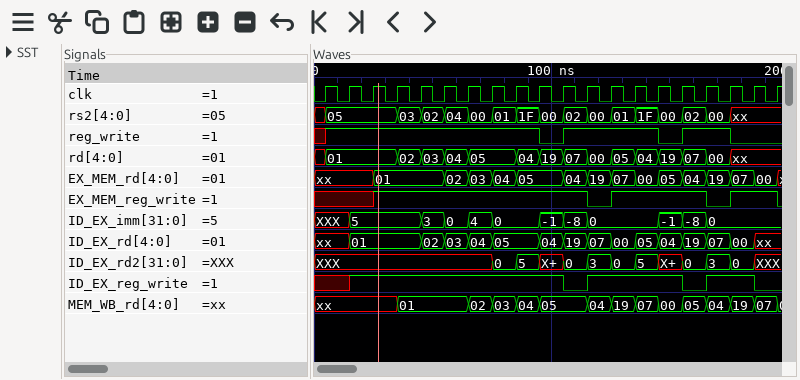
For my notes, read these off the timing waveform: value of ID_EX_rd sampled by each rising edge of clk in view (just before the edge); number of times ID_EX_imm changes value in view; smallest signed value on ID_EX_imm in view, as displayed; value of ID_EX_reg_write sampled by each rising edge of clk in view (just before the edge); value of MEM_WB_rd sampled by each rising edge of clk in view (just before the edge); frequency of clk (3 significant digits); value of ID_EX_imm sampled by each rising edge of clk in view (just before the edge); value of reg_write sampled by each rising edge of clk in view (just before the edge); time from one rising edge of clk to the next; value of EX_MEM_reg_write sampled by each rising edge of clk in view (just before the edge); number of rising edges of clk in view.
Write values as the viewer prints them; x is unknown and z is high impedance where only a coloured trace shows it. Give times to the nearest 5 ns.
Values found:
xx, xx, 01, 01, 01, 02, 03, 04, 05, 05, 04, 19, 07, 00, 05, 04, 19, 07, 00, xx
11
-8
x x 1 1 1 1 1 1 1 1 1 0 1 1 1 1 0 1 1 0
xx, xx, xx, xx, 01, 01, 01, 02, 03, 04, 05, 05, 04, 19, 07, 00, 05, 04, 19, 07
100 MHz
XXX, XXX, 5, 5, 5, 3, 0, 4, 0, 0, -1, -8, 0, 0, 0, -1, -8, 0, 0, 0
x 1 1 1 1 1 1 1 1 1 0 1 1 1 1 0 1 1 0 0
10 ns
x x x 1 1 1 1 1 1 1 1 1 0 1 1 1 1 0 1 1
20
